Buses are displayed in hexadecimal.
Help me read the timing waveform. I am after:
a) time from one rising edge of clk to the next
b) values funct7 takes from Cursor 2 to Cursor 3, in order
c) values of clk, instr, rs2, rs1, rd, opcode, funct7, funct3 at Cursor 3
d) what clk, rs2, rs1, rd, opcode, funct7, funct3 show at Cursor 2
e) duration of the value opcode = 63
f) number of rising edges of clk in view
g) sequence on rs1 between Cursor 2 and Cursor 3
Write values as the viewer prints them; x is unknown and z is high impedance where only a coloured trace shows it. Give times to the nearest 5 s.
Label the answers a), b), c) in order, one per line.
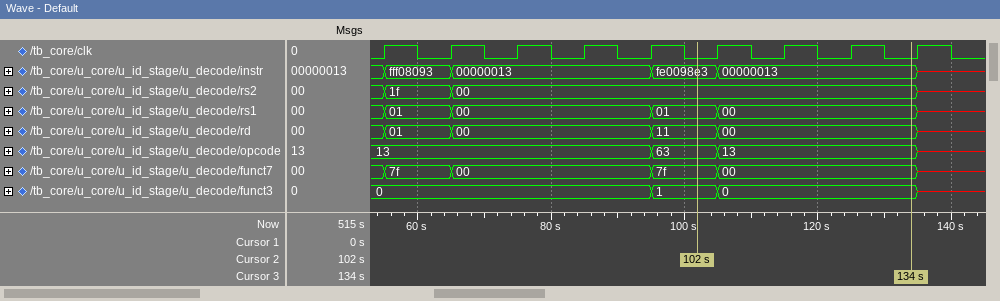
a) 10 s
b) 7f, 00
c) clk=0, instr=00000013, rs2=00, rs1=00, rd=00, opcode=13, funct7=00, funct3=0
d) clk=0, rs2=00, rs1=01, rd=11, opcode=63, funct7=7f, funct3=1
e) 10 s
f) 9
g) 01, 00
